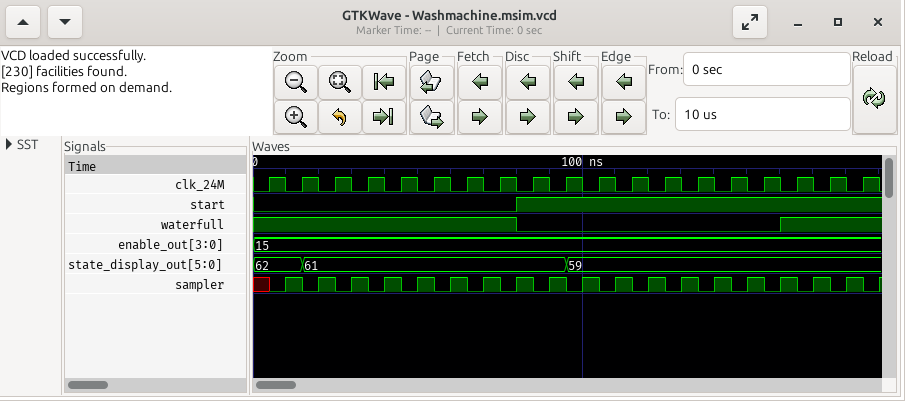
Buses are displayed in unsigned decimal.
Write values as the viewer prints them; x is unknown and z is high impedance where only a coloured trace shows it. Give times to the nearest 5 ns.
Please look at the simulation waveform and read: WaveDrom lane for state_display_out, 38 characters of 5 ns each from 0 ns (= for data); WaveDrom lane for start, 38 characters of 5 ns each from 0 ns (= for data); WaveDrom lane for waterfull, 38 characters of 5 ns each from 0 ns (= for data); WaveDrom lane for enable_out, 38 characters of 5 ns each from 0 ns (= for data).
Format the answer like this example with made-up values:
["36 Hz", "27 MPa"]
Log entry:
["{name: 'state_display_out', wave: '=..=...............=..................', data: '62 61 59'}", "{name: 'start', wave: '0...............1.....................'}", "{name: 'waterfull', wave: '1...............0...............1.....'}", "{name: 'enable_out', wave: '=.....................................', data: '15'}"]
